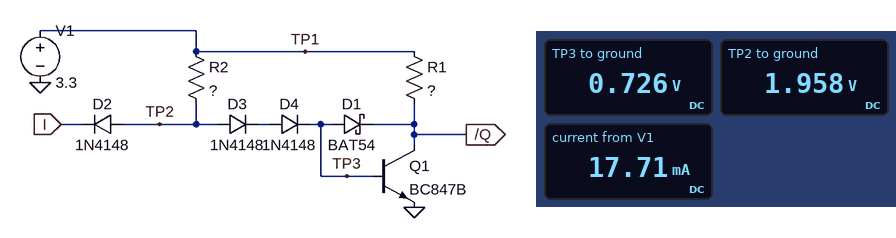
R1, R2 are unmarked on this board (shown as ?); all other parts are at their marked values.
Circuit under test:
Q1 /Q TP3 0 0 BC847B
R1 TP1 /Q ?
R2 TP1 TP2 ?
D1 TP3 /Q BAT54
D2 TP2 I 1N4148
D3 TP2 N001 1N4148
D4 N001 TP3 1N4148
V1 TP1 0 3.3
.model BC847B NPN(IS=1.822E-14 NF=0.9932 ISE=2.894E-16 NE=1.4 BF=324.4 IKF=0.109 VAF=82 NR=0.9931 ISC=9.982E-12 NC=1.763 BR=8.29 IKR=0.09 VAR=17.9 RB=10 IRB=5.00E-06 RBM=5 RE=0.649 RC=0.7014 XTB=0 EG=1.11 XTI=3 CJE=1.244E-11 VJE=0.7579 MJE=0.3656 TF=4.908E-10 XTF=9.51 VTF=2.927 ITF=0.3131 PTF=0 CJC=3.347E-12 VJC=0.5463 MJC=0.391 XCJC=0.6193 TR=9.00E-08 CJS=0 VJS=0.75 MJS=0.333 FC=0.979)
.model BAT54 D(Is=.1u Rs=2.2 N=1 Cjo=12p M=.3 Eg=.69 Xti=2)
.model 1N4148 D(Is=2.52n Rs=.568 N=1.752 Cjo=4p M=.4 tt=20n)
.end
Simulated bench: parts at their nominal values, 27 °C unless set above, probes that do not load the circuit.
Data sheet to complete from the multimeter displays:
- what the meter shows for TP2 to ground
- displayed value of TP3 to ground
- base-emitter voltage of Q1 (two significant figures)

1.958 V
0.726 V
730 mV
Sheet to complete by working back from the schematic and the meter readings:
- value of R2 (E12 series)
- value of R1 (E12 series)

680 Ω
180 Ω
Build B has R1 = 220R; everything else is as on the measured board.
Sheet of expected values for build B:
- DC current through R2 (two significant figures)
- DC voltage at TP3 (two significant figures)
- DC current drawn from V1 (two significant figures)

2.0 mA
720 mV
15 mA
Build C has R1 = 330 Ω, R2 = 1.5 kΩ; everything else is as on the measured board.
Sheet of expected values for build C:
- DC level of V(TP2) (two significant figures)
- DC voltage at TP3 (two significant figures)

1.9 V
700 mV
